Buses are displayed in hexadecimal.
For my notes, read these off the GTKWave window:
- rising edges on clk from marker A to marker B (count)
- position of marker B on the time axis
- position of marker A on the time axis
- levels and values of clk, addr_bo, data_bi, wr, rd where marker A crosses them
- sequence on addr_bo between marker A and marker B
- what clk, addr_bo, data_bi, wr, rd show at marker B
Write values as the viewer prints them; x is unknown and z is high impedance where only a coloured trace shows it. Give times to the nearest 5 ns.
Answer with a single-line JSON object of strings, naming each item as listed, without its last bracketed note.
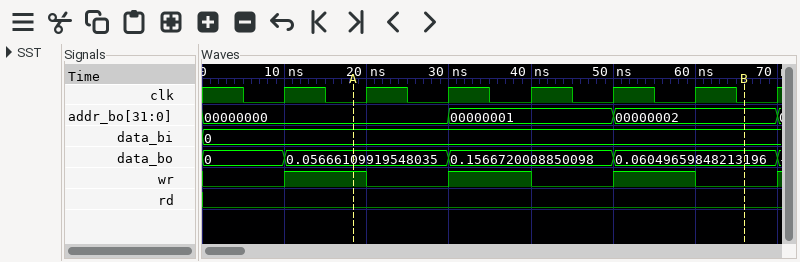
{"rising edges on clk from marker A to marker B": "5", "position of marker B on the time axis": "65 ns", "position of marker A on the time axis": "20 ns", "levels and values of clk, addr_bo, data_bi, wr, rd where marker A crosses them": "clk=0, addr_bo=00000000, data_bi=0, wr=1, rd=0", "sequence on addr_bo between marker A and marker B": "00000000, 00000001, 00000002", "what clk, addr_bo, data_bi, wr, rd show at marker B": "clk=0, addr_bo=00000002, data_bi=0, wr=0, rd=0"}
